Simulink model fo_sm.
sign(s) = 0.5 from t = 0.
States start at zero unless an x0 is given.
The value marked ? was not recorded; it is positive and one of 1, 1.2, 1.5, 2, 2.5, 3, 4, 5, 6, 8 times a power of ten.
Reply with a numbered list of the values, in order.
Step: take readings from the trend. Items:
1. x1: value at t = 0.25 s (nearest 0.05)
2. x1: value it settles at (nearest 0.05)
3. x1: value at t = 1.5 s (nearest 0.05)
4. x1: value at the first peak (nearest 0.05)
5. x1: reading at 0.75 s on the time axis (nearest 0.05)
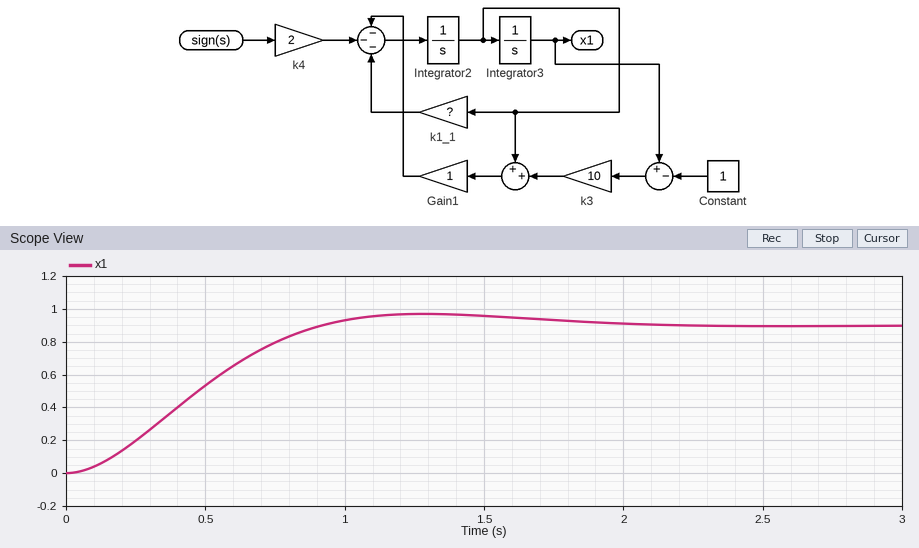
1. 0.20
2. 0.90
3. 0.95
4. 0.95
5. 0.80
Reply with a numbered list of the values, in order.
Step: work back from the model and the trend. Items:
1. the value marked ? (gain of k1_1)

1. 3
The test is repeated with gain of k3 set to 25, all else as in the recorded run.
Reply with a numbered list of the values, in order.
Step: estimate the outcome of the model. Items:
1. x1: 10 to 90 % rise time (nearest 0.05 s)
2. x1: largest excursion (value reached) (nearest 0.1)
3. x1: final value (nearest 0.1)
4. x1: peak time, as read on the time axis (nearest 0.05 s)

1. 0.30 s
2. 1.2
3. 1.0
4. 0.70 s
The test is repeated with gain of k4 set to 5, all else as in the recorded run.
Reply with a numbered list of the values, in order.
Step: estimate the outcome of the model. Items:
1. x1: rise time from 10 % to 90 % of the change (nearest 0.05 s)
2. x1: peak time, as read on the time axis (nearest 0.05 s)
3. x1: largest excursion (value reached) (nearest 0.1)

1. 0.60 s
2. 1.30 s
3. 0.8
